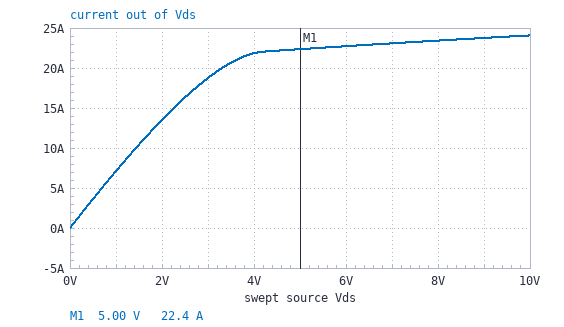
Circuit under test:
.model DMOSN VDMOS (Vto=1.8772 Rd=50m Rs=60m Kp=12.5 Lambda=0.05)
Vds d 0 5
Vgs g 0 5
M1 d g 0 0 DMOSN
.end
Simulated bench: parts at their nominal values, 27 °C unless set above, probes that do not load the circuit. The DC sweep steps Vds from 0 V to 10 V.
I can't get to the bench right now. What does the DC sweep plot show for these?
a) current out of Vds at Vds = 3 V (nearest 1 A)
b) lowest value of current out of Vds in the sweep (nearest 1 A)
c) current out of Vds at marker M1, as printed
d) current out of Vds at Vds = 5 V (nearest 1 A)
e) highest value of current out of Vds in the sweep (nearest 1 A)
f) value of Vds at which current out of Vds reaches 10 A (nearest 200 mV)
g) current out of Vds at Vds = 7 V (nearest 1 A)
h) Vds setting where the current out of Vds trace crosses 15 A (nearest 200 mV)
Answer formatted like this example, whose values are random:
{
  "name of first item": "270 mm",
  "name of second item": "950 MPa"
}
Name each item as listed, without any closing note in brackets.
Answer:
{
  "current out of Vds at Vds = 3 V": "19 A",
  "lowest value of current out of Vds in the sweep": "0 A",
  "current out of Vds at marker M1, as printed": "22.4 A",
  "current out of Vds at Vds = 5 V": "22 A",
  "highest value of current out of Vds in the sweep": "24 A",
  "value of Vds at which current out of Vds reaches 10 A": "1.4 V",
  "current out of Vds at Vds = 7 V": "23 A",
  "Vds setting where the current out of Vds trace crosses 15 A": "2.2 V"
}
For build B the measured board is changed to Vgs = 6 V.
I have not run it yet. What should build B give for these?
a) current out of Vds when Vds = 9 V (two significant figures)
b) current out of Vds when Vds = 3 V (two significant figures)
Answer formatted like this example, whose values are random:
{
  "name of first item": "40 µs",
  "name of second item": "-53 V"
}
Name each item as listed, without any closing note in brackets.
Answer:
{
  "current out of Vds when Vds = 9 V": "34 A",
  "current out of Vds when Vds = 3 V": "21 A"
}
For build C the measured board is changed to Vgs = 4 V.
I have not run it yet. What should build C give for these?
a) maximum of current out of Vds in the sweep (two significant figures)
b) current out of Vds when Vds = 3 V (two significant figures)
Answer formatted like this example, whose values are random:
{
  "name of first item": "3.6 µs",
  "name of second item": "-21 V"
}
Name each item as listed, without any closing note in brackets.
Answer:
{
  "maximum of current out of Vds in the sweep": "14 A",
  "current out of Vds when Vds = 3 V": "13 A"
}
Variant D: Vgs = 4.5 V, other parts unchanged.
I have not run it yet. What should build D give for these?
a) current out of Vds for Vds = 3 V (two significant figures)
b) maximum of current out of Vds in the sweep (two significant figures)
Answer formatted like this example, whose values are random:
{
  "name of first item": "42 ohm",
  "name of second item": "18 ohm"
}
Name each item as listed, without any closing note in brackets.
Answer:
{
  "current out of Vds for Vds = 3 V": "16 A",
  "maximum of current out of Vds in the sweep": "19 A"
}
